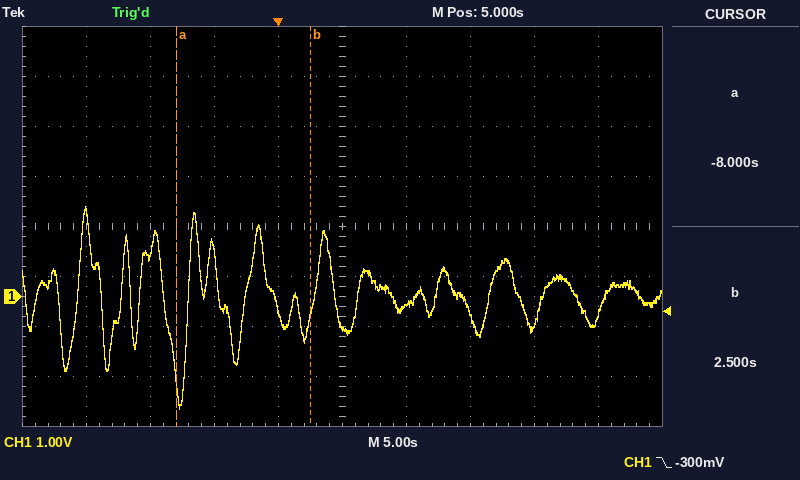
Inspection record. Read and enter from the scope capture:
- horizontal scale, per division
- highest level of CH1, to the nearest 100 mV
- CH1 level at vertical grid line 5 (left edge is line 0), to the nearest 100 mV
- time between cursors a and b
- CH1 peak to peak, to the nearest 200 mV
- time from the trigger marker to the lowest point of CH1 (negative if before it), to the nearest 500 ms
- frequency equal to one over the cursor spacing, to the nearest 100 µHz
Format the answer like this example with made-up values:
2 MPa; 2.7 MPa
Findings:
5 s; 1.8 V; -600 mV; 10.5 s; 4.0 V; -7.5 s; 95.2 mHz
